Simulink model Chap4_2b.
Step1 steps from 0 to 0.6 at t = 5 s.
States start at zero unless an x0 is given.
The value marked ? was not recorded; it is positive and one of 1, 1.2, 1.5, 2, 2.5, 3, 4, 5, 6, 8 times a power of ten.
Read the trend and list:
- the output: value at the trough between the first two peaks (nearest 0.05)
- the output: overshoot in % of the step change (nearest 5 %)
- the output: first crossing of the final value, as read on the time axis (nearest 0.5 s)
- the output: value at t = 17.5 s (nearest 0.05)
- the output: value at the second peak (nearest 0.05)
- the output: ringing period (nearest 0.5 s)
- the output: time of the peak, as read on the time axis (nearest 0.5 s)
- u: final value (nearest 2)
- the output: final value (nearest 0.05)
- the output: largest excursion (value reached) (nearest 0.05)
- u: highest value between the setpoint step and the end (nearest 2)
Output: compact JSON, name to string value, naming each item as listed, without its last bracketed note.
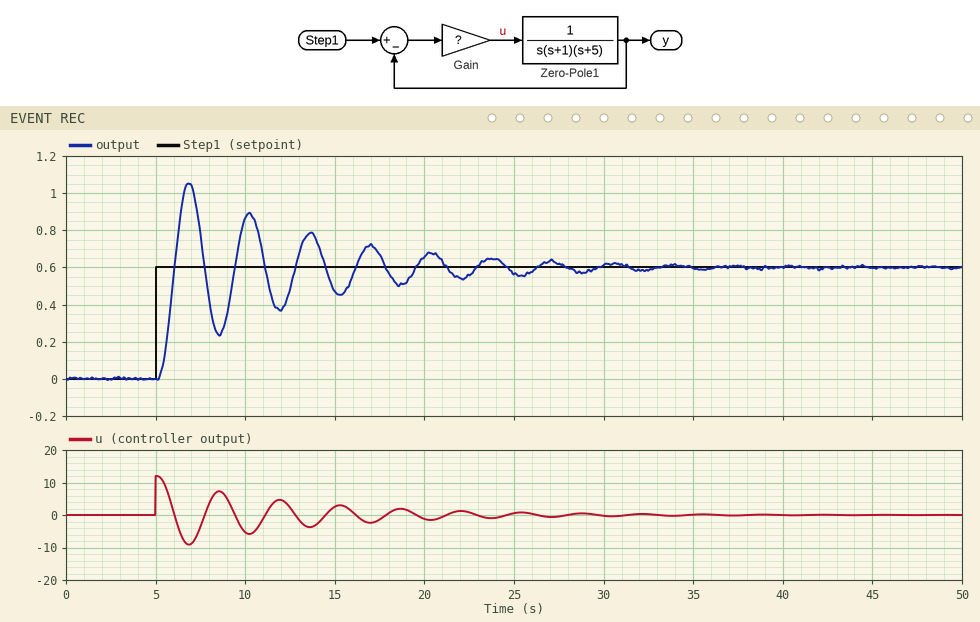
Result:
{"the output: value at the trough between the first two peaks": "0.25", "the output: overshoot in % of the step change": "75 %", "the output: first crossing of the final value, as read on the time axis": "6.0 s", "the output: value at t = 17.5 s": "0.65", "the output: value at the second peak": "0.90", "the output: ringing period": "3.5 s", "the output: time of the peak, as read on the time axis": "7.0 s", "u: final value": "0", "the output: final value": "0.60", "the output: largest excursion (value reached)": "1.05", "u: highest value between the setpoint step and the end": "12"}
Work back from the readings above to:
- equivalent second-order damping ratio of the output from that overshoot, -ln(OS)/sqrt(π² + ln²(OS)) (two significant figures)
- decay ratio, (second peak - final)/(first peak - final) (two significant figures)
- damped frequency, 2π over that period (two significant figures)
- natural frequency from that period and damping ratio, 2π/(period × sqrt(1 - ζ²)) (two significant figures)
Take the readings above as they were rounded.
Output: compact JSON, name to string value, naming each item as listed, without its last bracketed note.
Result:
{"equivalent second-order damping ratio of the output from that overshoot, -ln(OS)/sqrt(π² + ln²(OS))": "0.091", "decay ratio, (second peak - final)/(first peak - final)": "0.67", "damped frequency, 2π over that period": "1.8 rad/s", "natural frequency from that period and damping ratio, 2π/(period × sqrt(1 - ζ²))": "1.8 rad/s"}
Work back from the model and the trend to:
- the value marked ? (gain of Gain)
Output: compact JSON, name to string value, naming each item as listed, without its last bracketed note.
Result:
{"the value marked ?": "20"}
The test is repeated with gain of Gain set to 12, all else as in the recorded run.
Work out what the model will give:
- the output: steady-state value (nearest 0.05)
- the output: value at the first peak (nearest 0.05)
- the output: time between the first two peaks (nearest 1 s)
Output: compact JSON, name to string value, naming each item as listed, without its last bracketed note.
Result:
{"the output: steady-state value": "0.60", "the output: value at the first peak": "0.95", "the output: time between the first two peaks": "4 s"}
